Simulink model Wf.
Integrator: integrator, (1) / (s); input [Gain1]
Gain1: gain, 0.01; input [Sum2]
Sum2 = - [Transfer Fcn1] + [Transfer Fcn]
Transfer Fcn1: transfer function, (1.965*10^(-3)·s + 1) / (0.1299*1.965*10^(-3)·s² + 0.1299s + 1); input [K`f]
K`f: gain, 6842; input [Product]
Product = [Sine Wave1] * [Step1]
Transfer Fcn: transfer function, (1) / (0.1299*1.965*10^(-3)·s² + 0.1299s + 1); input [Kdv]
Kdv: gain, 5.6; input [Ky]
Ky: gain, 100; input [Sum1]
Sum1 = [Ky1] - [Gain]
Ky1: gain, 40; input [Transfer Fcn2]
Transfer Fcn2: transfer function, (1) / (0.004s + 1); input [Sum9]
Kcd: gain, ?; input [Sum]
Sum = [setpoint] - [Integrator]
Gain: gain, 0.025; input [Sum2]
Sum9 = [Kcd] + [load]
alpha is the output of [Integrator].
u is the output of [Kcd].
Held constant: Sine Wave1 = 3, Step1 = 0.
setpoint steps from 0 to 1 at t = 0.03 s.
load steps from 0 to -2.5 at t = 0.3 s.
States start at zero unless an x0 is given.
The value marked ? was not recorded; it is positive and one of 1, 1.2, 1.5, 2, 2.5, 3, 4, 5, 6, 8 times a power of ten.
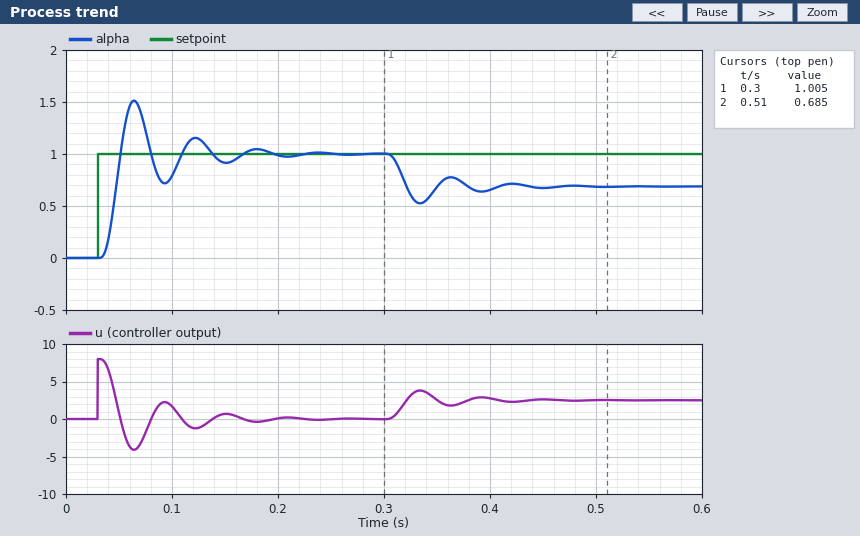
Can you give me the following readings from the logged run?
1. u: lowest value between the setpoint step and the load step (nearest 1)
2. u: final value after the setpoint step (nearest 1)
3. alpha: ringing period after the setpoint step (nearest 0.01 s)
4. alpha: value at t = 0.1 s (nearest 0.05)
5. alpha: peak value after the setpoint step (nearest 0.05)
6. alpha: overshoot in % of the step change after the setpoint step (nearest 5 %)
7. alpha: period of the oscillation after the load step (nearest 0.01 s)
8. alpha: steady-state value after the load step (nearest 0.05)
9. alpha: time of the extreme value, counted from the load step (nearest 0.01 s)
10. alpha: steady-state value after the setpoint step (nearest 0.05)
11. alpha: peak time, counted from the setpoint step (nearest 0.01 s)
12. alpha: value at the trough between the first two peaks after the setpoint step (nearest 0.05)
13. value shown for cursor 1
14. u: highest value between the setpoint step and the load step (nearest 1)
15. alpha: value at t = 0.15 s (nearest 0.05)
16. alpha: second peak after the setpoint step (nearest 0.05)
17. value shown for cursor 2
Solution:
-4
0
0.06 s
0.80
1.50
50 %
0.06 s
0.70
0.03 s
1.00
0.03 s
0.70
1.005
8
0.90
1.15
0.685
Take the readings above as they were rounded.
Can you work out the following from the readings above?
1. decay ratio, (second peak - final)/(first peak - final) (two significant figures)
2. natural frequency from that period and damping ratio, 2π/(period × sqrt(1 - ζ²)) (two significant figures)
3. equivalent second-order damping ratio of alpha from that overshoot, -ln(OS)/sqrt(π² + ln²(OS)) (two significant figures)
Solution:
0.30
110 rad/s
0.22
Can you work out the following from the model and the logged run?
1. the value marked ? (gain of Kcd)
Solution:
8
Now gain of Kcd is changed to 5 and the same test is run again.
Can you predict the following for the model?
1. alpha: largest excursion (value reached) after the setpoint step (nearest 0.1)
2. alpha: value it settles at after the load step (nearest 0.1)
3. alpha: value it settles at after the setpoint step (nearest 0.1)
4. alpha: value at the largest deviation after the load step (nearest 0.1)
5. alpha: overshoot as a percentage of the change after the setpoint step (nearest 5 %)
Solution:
1.3
0.5
1.0
0.4
25 %
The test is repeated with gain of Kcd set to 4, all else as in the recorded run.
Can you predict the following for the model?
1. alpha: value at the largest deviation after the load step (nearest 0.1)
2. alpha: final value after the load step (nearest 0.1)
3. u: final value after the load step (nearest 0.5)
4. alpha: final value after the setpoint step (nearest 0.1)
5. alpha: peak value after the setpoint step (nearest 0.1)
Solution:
0.3
0.4
2.5
1.0
1.2
